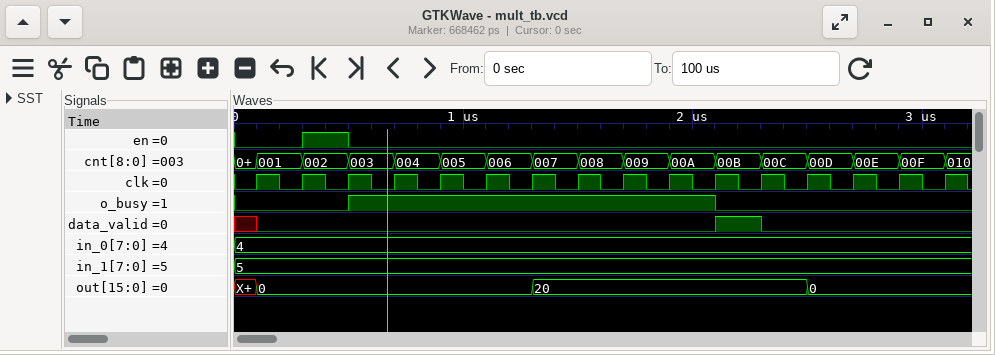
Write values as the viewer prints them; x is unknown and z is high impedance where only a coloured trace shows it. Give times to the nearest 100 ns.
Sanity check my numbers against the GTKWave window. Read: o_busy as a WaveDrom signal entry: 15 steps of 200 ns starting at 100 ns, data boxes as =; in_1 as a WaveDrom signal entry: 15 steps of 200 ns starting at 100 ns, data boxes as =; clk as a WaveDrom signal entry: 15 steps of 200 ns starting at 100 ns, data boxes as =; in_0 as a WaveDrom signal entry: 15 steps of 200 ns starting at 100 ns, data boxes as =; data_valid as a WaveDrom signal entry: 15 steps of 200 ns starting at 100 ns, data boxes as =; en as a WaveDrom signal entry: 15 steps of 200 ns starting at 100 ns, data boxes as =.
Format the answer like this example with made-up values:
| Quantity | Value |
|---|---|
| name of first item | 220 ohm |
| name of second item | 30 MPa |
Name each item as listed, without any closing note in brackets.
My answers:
| Quantity | Value |
|---|---|
| o_busy as a WaveDrom signal entry: 15 steps of 200 ns starting at 100 ns, data boxes as = | {name: 'o_busy', wave: '0.1.......0....'} |
| in_1 as a WaveDrom signal entry: 15 steps of 200 ns starting at 100 ns, data boxes as = | {name: 'in_1', wave: '=..............', data: '5'} |
| clk as a WaveDrom signal entry: 15 steps of 200 ns starting at 100 ns, data boxes as = | {name: 'clk', wave: 'p..............'} |
| in_0 as a WaveDrom signal entry: 15 steps of 200 ns starting at 100 ns, data boxes as = | {name: 'in_0', wave: '=..............', data: '4'} |
| data_valid as a WaveDrom signal entry: 15 steps of 200 ns starting at 100 ns, data boxes as = | {name: 'data_valid', wave: '0.........10...'} |
| en as a WaveDrom signal entry: 15 steps of 200 ns starting at 100 ns, data boxes as = | {name: 'en', wave: '010............'} |
